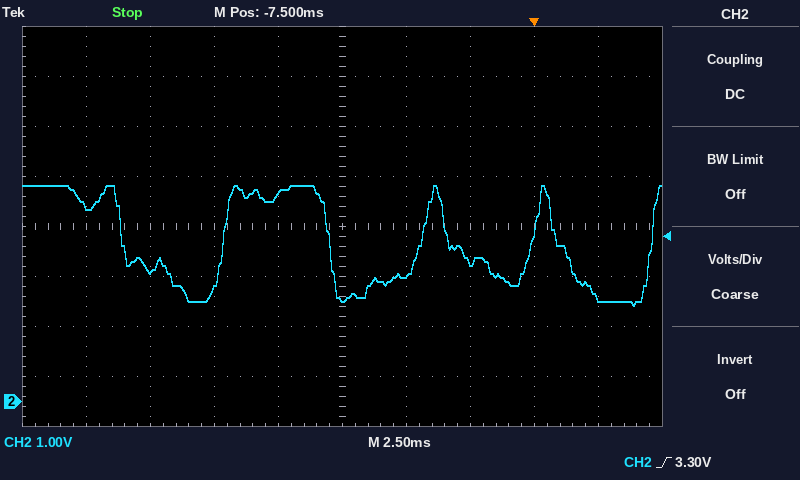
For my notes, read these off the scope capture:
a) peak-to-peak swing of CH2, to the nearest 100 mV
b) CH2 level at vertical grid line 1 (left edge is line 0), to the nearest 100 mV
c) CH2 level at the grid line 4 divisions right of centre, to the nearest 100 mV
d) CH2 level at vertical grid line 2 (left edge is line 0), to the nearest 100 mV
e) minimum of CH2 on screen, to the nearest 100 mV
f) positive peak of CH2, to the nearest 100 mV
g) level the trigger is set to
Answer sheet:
2.4 V
3.9 V
2.1 V
2.6 V
1.9 V
4.3 V
3.30 V
